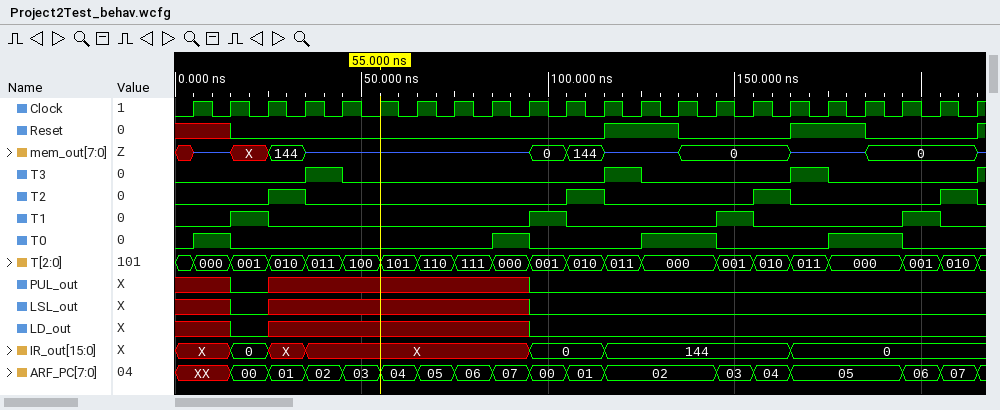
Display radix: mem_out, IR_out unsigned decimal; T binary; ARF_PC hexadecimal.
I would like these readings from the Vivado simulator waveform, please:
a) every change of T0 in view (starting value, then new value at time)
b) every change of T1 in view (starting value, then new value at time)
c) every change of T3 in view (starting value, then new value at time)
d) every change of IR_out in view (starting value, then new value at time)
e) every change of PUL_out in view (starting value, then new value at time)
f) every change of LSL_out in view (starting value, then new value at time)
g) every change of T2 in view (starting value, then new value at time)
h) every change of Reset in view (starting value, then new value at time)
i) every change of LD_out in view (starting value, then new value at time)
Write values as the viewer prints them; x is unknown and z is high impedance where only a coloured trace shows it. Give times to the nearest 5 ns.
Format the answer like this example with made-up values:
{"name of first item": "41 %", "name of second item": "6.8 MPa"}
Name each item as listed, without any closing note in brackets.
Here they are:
{"every change of T0 in view": "0, 1 at 5 ns, 0 at 15 ns, 1 at 85 ns, 0 at 95 ns, 1 at 125 ns, 0 at 145 ns, 1 at 175 ns, 0 at 195 ns", "every change of T1 in view": "0, 1 at 15 ns, 0 at 25 ns, 1 at 95 ns, 0 at 105 ns, 1 at 145 ns, 0 at 155 ns, 1 at 195 ns, 0 at 205 ns", "every change of T3 in view": "0, 1 at 35 ns, 0 at 45 ns, 1 at 115 ns, 0 at 125 ns, 1 at 165 ns, 0 at 175 ns, 1 at 215 ns", "every change of IR_out in view": "X, 0 at 15 ns, X at 25 ns, X at 35 ns, 0 at 95 ns, 144 at 115 ns, 0 at 165 ns", "every change of PUL_out in view": "x, 0 at 15 ns, x at 25 ns, 0 at 95 ns", "every change of LSL_out in view": "x, 0 at 15 ns, x at 25 ns, 0 at 95 ns", "every change of T2 in view": "0, 1 at 25 ns, 0 at 35 ns, 1 at 105 ns, 0 at 115 ns, 1 at 155 ns, 0 at 165 ns, 1 at 205 ns, 0 at 215 ns", "every change of Reset in view": "x, 0 at 15 ns, 1 at 115 ns, 0 at 135 ns, 1 at 165 ns, 0 at 185 ns, 1 at 215 ns", "every change of LD_out in view": "x, 0 at 15 ns, x at 25 ns, 0 at 95 ns"}
